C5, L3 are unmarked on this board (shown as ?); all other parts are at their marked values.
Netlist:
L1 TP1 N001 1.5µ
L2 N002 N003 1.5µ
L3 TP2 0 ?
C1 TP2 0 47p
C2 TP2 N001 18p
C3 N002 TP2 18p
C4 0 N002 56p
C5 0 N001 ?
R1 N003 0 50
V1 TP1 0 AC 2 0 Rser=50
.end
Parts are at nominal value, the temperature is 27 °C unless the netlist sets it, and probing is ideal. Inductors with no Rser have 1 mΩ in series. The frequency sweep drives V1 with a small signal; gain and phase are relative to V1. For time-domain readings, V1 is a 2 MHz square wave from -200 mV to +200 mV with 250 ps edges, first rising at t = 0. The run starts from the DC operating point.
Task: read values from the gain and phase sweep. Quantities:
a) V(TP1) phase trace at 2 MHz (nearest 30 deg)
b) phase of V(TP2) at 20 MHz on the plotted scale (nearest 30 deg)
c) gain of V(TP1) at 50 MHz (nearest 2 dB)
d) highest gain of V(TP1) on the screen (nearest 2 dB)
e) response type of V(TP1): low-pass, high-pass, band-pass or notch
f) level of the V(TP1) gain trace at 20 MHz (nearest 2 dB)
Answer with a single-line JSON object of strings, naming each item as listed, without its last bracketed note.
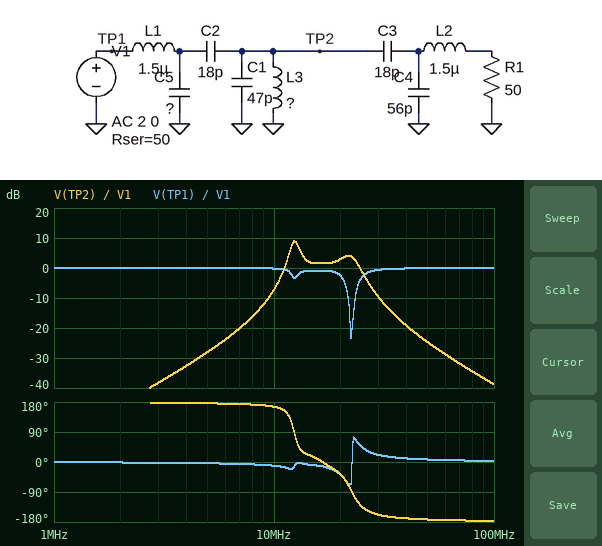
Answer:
{"V(TP1) phase trace at 2 MHz": "0 deg", "phase of V(TP2) at 20 MHz on the plotted scale": "-30 deg", "gain of V(TP1) at 50 MHz": "0 dB", "highest gain of V(TP1) on the screen": "0 dB", "response type of V(TP1): low-pass, high-pass, band-pass or notch": "notch", "level of the V(TP1) gain trace at 20 MHz": "-2 dB"}
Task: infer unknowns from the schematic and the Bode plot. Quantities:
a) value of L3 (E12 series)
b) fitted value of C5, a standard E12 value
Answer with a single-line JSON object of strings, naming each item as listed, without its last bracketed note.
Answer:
{"value of L3": "1.8 µH", "fitted value of C5, a standard E12 value": "22 pF"}
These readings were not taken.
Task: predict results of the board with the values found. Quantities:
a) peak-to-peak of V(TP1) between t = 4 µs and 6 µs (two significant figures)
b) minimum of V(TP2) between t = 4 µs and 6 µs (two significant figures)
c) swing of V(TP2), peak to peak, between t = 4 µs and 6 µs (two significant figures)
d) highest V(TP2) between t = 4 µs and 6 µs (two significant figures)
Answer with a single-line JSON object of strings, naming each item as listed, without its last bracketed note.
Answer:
{"peak-to-peak of V(TP1) between t = 4 µs and 6 µs": "490 mV", "minimum of V(TP2) between t = 4 µs and 6 µs": "-150 mV", "swing of V(TP2), peak to peak, between t = 4 µs and 6 µs": "300 mV", "highest V(TP2) between t = 4 µs and 6 µs": "150 mV"}
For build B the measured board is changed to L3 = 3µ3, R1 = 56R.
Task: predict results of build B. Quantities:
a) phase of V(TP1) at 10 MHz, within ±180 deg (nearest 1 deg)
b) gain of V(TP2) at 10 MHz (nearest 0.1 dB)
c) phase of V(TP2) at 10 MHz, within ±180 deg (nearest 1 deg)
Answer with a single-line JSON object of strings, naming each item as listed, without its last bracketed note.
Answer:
{"phase of V(TP1) at 10 MHz, within ±180 deg": "-1 deg", "gain of V(TP2) at 10 MHz": "6.1 dB", "phase of V(TP2) at 10 MHz, within ±180 deg": "15 deg"}
